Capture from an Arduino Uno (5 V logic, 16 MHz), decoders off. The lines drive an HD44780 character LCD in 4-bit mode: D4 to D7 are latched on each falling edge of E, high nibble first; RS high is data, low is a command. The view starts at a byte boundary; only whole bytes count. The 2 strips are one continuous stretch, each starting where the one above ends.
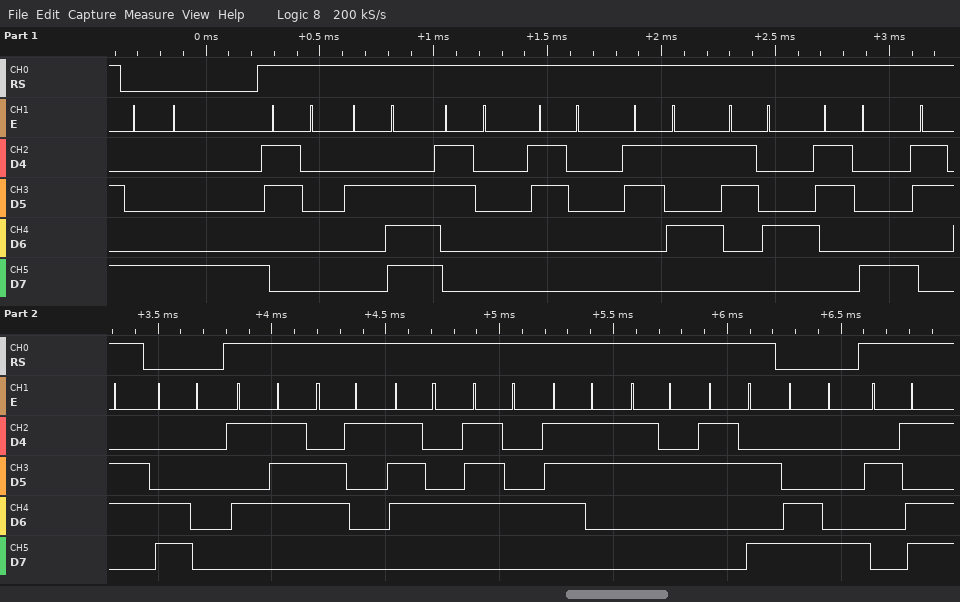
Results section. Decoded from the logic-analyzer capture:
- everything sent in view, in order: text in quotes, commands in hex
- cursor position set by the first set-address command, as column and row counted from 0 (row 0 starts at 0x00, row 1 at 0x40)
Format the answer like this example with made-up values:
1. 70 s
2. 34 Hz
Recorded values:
1. 0x88 "0.005486" 0xC0 "Watts2:" 0xC8 "-"
2. column 8, row 0
